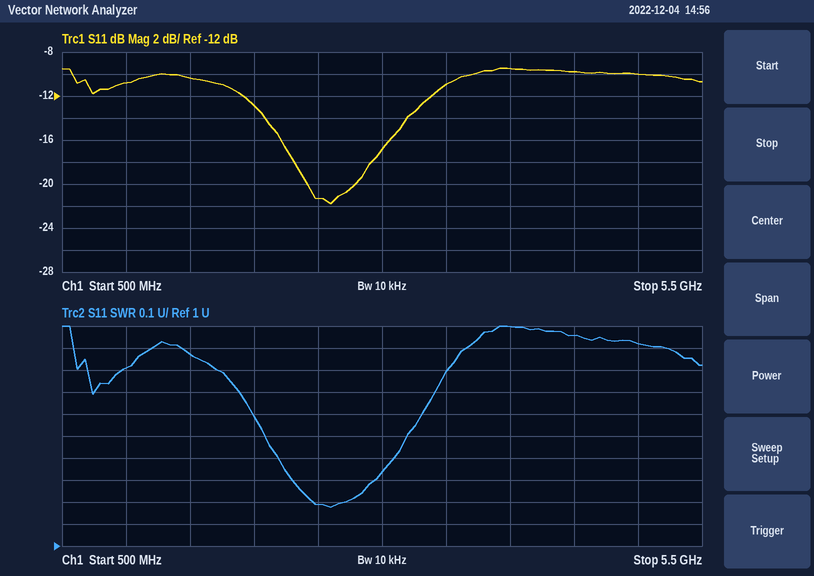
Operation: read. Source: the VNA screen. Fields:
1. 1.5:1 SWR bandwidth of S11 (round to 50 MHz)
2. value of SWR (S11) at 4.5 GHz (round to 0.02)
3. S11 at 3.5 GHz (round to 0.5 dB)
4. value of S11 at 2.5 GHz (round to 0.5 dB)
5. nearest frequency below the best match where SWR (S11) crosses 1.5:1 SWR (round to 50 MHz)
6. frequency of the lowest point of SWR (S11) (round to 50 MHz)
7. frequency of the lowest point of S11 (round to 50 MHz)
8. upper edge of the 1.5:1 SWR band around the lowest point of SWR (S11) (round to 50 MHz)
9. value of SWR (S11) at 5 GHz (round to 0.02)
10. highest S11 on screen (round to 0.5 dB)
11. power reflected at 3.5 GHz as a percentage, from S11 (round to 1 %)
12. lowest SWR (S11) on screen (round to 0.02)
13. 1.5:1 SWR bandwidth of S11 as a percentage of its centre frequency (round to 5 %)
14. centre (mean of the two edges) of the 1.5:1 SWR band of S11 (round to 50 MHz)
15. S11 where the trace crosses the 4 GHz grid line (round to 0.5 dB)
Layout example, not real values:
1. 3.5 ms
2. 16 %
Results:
1. 1.10 GHz
2. 1.96
3. -11.0 dB
4. -21.5 dB
5. 2.10 GHz
6. 2.60 GHz
7. 2.60 GHz
8. 3.20 GHz
9. 1.92
10. -9.5 dB
11. 8 %
12. 1.18
13. 40 %
14. 2.65 GHz
15. -9.5 dB
